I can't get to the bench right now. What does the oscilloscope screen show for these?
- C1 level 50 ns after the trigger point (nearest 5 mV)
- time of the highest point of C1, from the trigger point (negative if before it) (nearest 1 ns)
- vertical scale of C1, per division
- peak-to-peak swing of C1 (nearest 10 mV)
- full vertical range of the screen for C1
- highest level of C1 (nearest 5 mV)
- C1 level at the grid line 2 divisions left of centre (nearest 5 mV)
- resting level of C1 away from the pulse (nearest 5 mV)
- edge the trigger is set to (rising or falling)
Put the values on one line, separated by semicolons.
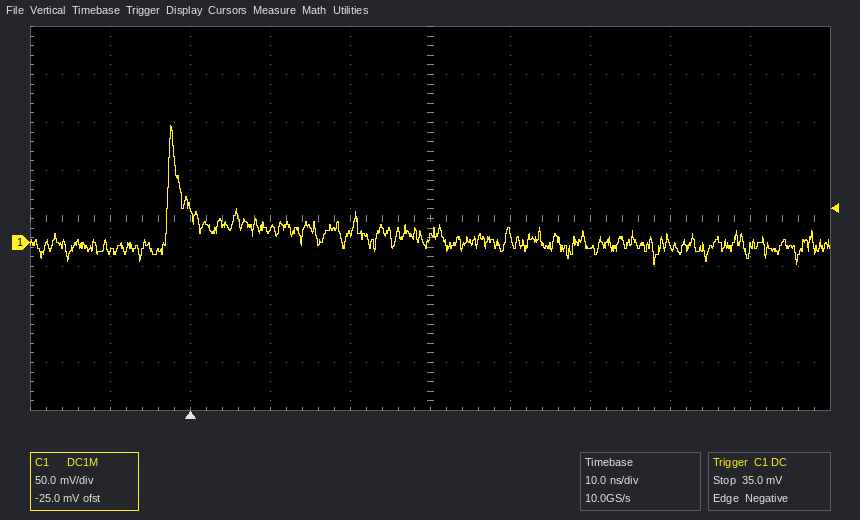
-5 mV; -2 ns; 50 mV; 140 mV; 400 mV; 120 mV; 15 mV; 0 mV; falling
